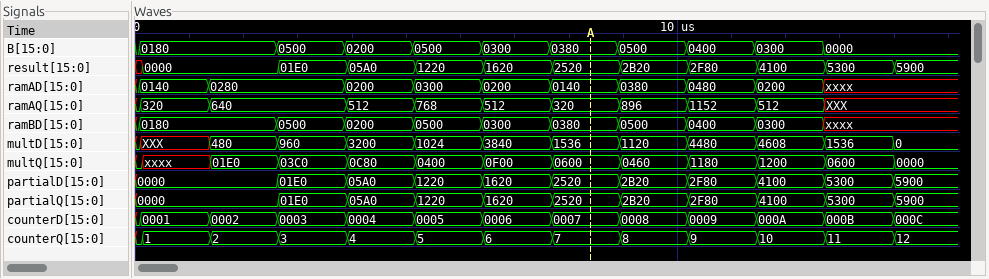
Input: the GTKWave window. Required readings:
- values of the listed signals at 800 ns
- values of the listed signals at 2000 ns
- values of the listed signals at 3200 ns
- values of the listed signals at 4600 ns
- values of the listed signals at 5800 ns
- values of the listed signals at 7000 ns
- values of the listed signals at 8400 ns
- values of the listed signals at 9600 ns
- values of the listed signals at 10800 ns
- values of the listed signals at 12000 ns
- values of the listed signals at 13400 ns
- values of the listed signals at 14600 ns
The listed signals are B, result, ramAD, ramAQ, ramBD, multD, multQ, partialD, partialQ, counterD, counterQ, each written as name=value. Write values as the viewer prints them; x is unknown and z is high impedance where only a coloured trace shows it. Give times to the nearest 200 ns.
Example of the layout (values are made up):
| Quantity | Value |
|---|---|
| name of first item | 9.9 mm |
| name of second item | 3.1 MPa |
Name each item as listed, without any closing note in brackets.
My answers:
| Quantity | Value |
|---|---|
| values of the listed signals at 800 ns | B=0180, result=0000, ramAD=0140, ramAQ=320, ramBD=0180, multD=XXX, multQ=xxxx, partialD=0000, partialQ=0000, counterD=0001, counterQ=1 |
| values of the listed signals at 2000 ns | B=0180, result=0000, ramAD=0280, ramAQ=640, ramBD=0180, multD=480, multQ=01E0, partialD=0000, partialQ=0000, counterD=0002, counterQ=2 |
| values of the listed signals at 3200 ns | B=0500, result=01E0, ramAD=0280, ramAQ=640, ramBD=0500, multD=960, multQ=03C0, partialD=01E0, partialQ=01E0, counterD=0003, counterQ=3 |
| values of the listed signals at 4600 ns | B=0200, result=05A0, ramAD=0200, ramAQ=512, ramBD=0200, multD=3200, multQ=0C80, partialD=05A0, partialQ=05A0, counterD=0004, counterQ=4 |
| values of the listed signals at 5800 ns | B=0500, result=1220, ramAD=0300, ramAQ=768, ramBD=0500, multD=1024, multQ=0400, partialD=1220, partialQ=1220, counterD=0005, counterQ=5 |
| values of the listed signals at 7000 ns | B=0300, result=1620, ramAD=0200, ramAQ=512, ramBD=0300, multD=3840, multQ=0F00, partialD=1620, partialQ=1620, counterD=0006, counterQ=6 |
| values of the listed signals at 8400 ns | B=0380, result=2520, ramAD=0140, ramAQ=320, ramBD=0380, multD=1536, multQ=0600, partialD=2520, partialQ=2520, counterD=0007, counterQ=7 |
| values of the listed signals at 9600 ns | B=0500, result=2B20, ramAD=0380, ramAQ=896, ramBD=0500, multD=1120, multQ=0460, partialD=2B20, partialQ=2B20, counterD=0008, counterQ=8 |
| values of the listed signals at 10800 ns | B=0400, result=2F80, ramAD=0480, ramAQ=1152, ramBD=0400, multD=4480, multQ=1180, partialD=2F80, partialQ=2F80, counterD=0009, counterQ=9 |
| values of the listed signals at 12000 ns | B=0300, result=4100, ramAD=0200, ramAQ=512, ramBD=0300, multD=4608, multQ=1200, partialD=4100, partialQ=4100, counterD=000A, counterQ=10 |
| values of the listed signals at 13400 ns | B=0000, result=5300, ramAD=xxxx, ramAQ=XXX, ramBD=xxxx, multD=1536, multQ=0600, partialD=5300, partialQ=5300, counterD=000B, counterQ=11 |
| values of the listed signals at 14600 ns | B=0000, result=5900, ramAD=xxxx, ramAQ=XXX, ramBD=xxxx, multD=0, multQ=0000, partialD=5900, partialQ=5900, counterD=000C, counterQ=12 |
